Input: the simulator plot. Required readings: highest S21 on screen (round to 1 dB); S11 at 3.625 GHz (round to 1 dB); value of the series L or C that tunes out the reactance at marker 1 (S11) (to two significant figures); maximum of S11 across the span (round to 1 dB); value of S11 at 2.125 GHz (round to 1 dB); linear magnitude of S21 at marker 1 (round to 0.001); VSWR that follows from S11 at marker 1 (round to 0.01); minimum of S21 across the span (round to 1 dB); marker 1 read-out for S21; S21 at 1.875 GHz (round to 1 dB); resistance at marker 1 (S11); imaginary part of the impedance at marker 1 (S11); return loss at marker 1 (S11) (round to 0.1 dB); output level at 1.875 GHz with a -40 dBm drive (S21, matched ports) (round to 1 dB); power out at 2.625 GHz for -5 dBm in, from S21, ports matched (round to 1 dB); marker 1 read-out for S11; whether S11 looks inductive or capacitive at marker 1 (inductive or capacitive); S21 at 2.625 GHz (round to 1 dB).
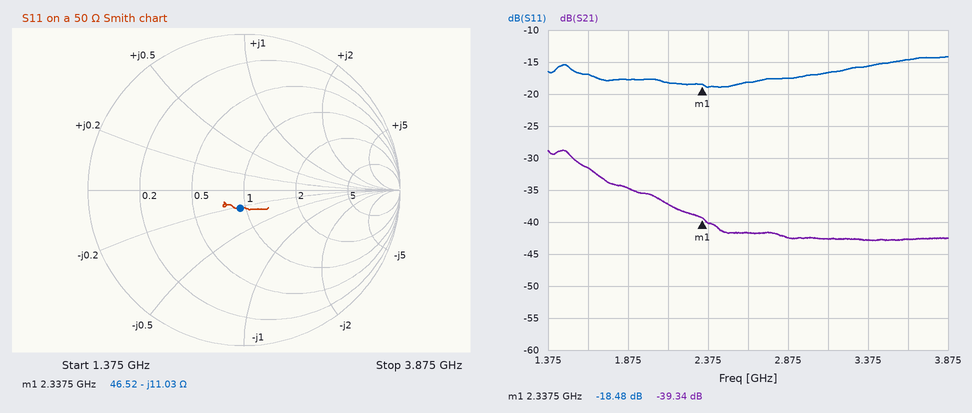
-29 dB
-15 dB
750 pH
-14 dB
-18 dB
0.011
1.27
-43 dB
-39.34 dB
-35 dB
46.52 Ω
-11.03 Ω
18.5 dB
-75 dBm
-47 dBm
-18.48 dB
capacitive
-42 dB
